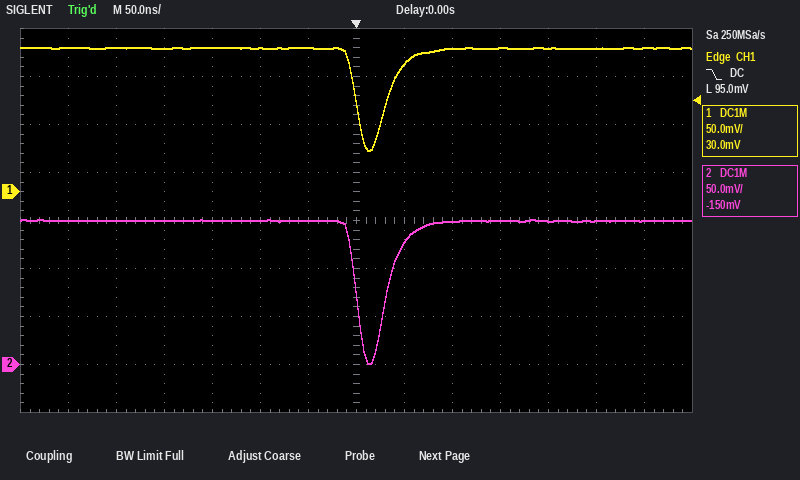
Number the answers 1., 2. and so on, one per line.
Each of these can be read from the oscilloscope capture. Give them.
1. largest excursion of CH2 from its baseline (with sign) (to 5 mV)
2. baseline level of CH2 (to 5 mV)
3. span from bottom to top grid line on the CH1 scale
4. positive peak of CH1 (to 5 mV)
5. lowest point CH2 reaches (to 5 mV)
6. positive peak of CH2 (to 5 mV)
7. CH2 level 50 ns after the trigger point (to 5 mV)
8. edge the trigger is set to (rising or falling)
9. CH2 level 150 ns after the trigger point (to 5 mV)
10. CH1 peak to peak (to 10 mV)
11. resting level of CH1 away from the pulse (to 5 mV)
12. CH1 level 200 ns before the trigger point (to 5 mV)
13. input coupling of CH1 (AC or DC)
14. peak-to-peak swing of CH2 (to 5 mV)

1. -150 mV
2. 150 mV
3. 400 mV
4. 150 mV
5. 0 mV
6. 150 mV
7. 125 mV
8. falling
9. 150 mV
10. 110 mV
11. 150 mV
12. 150 mV
13. DC
14. 150 mV
